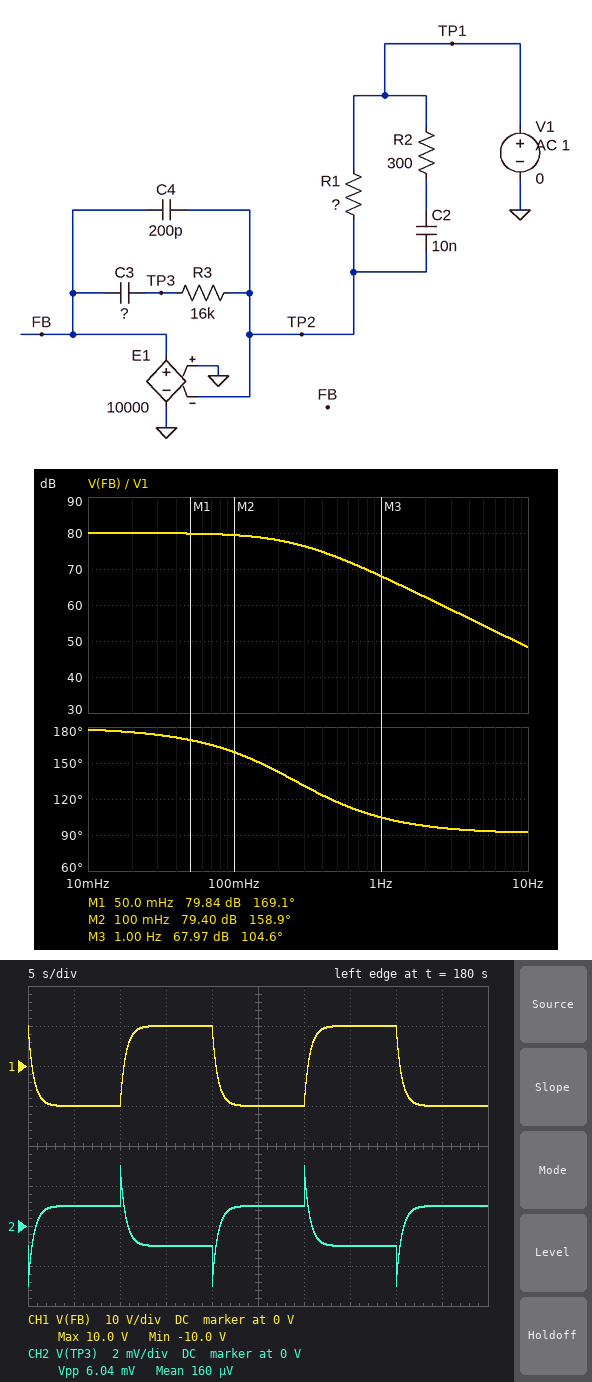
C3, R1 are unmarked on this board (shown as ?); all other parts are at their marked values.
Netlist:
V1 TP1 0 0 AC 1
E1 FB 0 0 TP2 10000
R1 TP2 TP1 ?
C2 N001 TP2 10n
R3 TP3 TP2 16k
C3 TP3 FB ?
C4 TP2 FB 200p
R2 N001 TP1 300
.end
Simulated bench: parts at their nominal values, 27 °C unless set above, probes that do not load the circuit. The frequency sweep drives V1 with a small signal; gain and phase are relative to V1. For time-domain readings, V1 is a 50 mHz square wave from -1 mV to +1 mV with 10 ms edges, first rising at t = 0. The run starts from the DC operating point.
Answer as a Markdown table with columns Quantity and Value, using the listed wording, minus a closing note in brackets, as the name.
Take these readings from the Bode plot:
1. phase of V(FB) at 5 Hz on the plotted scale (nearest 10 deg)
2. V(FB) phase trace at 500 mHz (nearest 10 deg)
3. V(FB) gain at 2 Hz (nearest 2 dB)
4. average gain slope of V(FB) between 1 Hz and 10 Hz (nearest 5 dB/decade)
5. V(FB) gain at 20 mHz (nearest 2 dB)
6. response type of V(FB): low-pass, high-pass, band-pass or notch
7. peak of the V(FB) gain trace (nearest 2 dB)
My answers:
| Quantity | Value |
|---|---|
| phase of V(FB) at 5 Hz on the plotted scale | 90 deg |
| V(FB) phase trace at 500 mHz | 120 deg |
| V(FB) gain at 2 Hz | 62 dB |
| average gain slope of V(FB) between 1 Hz and 10 Hz | -20 dB/decade |
| V(FB) gain at 20 mHz | 80 dB |
| response type of V(FB): low-pass, high-pass, band-pass or notch | low-pass |
| peak of the V(FB) gain trace | 80 dB |
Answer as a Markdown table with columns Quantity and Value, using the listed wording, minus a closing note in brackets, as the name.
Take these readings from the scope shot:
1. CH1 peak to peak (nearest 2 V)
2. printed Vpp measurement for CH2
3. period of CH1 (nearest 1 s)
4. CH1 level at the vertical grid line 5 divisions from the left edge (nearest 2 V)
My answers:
| Quantity | Value |
|---|---|
| CH1 peak to peak | 20 V |
| printed Vpp measurement for CH2 | 6.04 mV |
| period of CH1 | 20 s |
| CH1 level at the vertical grid line 5 divisions from the left edge | -10 V |
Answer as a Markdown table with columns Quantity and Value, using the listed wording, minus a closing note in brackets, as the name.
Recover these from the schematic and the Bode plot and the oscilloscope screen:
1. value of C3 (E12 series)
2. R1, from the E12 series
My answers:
| Quantity | Value |
|---|---|
| value of C3 | 3.9 nF |
| R1, from the E12 series | 15 kΩ |
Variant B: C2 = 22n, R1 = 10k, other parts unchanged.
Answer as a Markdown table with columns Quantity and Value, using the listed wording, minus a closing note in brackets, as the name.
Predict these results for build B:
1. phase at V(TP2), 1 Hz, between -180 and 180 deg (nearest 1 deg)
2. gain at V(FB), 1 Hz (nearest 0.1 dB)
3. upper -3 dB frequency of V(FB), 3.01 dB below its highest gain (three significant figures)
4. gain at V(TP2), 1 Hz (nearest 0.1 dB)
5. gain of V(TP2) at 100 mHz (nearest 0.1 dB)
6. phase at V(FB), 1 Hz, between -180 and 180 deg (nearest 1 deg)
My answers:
| Quantity | Value |
|---|---|
| phase at V(TP2), 1 Hz, between -180 and 180 deg | -69 deg |
| gain at V(FB), 1 Hz | 71.2 dB |
| upper -3 dB frequency of V(FB), 3.01 dB below its highest gain | 388 mHz |
| gain at V(TP2), 1 Hz | -8.8 dB |
| gain of V(TP2) at 100 mHz | -0.3 dB |
| phase at V(FB), 1 Hz, between -180 and 180 deg | 111 deg |
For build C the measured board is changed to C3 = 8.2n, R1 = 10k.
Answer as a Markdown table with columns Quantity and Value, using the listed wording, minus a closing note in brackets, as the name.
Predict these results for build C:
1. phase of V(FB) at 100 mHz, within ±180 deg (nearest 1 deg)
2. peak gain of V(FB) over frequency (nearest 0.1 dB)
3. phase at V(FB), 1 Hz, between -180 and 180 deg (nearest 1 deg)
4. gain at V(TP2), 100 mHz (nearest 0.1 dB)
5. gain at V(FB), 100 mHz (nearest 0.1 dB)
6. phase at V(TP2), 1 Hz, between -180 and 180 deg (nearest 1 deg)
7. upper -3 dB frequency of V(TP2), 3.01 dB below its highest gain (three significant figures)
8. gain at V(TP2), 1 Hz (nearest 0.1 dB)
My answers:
| Quantity | Value |
|---|---|
| phase of V(FB) at 100 mHz, within ±180 deg | 152 deg |
| peak gain of V(FB) over frequency | 80.0 dB |
| phase at V(FB), 1 Hz, between -180 and 180 deg | 101 deg |
| gain at V(TP2), 100 mHz | -1.1 dB |
| gain at V(FB), 100 mHz | 78.9 dB |
| phase at V(TP2), 1 Hz, between -180 and 180 deg | -79 deg |
| upper -3 dB frequency of V(TP2), 3.01 dB below its highest gain | 189 mHz |
| gain at V(TP2), 1 Hz | -14.6 dB |
